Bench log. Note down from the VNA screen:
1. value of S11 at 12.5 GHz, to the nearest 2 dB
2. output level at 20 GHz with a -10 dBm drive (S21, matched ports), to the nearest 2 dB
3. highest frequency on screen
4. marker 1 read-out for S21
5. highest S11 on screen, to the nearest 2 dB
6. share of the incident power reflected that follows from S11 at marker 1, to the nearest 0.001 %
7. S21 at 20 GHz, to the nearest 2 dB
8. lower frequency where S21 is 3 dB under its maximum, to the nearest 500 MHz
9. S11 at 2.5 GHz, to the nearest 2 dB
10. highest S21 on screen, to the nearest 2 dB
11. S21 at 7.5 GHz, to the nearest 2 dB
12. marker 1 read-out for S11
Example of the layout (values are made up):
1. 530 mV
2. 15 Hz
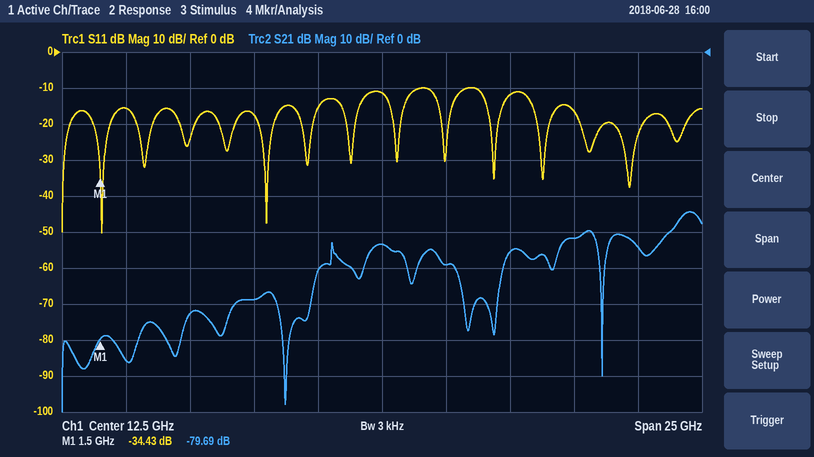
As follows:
1. -12 dB
2. -62 dBm
3. 25 GHz
4. -79.69 dB
5. -10 dB
6. 0.036 %
7. -52 dB
8. 24.0 GHz
9. -16 dB
10. -44 dB
11. -68 dB
12. -34.43 dB
